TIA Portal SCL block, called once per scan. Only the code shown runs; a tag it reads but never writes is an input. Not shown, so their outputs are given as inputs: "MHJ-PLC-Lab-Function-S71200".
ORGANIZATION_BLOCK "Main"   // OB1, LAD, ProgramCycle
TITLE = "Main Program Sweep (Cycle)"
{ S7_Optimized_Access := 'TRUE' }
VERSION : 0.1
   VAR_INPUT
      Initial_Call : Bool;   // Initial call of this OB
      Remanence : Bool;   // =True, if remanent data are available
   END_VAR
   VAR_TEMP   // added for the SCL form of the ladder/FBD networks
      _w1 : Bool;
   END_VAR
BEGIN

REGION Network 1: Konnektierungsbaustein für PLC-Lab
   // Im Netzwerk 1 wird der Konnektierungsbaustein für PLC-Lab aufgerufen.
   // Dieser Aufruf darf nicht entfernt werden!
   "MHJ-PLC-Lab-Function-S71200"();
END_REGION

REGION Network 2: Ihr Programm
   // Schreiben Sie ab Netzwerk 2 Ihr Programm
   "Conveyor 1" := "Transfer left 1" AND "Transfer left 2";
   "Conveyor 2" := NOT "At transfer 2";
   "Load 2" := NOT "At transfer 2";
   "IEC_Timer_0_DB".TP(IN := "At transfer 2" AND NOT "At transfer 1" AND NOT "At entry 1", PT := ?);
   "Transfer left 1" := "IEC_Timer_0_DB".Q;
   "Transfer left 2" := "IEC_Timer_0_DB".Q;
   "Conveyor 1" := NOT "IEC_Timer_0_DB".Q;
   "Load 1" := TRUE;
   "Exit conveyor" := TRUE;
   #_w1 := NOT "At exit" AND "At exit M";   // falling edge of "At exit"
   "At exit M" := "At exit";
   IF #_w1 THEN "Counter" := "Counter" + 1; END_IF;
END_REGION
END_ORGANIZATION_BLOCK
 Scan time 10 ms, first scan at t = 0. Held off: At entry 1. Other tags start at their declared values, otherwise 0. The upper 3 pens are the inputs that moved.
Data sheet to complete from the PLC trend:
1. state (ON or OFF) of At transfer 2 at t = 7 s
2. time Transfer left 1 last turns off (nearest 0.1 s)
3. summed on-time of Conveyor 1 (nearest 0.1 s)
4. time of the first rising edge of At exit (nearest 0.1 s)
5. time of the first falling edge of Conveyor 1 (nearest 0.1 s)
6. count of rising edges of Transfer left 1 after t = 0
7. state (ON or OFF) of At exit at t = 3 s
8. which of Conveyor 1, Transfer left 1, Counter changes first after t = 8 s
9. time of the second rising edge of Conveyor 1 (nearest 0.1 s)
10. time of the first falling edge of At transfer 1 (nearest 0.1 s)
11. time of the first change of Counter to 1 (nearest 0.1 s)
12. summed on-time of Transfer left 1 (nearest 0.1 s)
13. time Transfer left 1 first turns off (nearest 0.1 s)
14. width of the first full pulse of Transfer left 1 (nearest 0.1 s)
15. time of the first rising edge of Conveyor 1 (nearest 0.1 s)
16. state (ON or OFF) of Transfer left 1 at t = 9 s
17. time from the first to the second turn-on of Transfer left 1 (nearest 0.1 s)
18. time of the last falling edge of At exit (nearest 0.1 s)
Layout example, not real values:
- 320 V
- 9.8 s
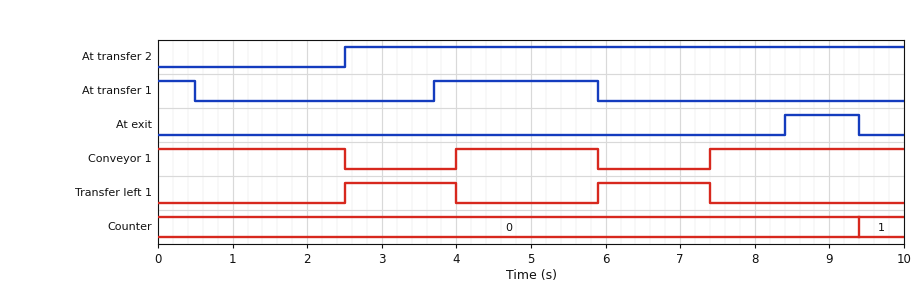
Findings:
- ON
- 7.4 s
- 7.0 s
- 8.4 s
- 2.5 s
- 2
- OFF
- Counter
- 7.4 s
- 0.5 s
- 9.4 s
- 3.0 s
- 4.0 s
- 1.5 s
- 4.0 s
- OFF
- 3.4 s
- 9.4 s
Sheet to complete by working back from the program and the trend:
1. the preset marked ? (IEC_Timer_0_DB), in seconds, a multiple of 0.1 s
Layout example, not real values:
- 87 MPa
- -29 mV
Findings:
- 1.5 s
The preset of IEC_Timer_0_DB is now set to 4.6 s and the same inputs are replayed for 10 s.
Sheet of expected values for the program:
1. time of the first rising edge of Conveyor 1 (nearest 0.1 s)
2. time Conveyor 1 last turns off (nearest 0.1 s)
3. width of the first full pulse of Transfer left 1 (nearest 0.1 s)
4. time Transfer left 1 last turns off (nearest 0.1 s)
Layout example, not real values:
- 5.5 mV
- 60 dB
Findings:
- 7.1 s
- 2.5 s
- 4.6 s
- 7.1 s
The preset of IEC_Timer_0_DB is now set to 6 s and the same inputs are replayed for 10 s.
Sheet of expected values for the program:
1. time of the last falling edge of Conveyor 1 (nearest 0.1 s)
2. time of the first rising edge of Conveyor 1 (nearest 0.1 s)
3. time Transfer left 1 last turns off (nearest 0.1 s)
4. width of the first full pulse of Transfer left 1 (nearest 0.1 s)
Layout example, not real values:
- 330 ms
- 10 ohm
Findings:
- 2.5 s
- 8.5 s
- 8.5 s
- 6.0 s
